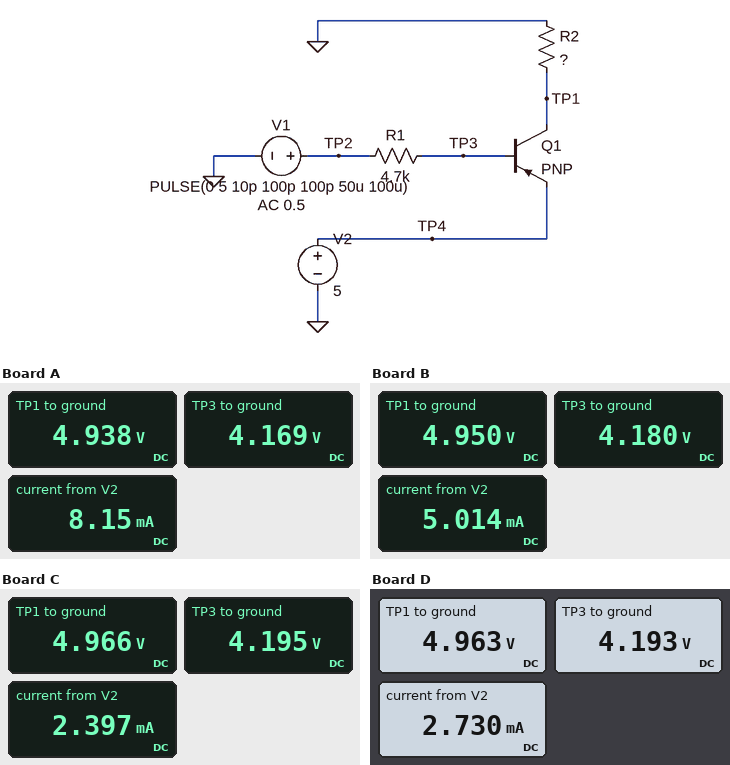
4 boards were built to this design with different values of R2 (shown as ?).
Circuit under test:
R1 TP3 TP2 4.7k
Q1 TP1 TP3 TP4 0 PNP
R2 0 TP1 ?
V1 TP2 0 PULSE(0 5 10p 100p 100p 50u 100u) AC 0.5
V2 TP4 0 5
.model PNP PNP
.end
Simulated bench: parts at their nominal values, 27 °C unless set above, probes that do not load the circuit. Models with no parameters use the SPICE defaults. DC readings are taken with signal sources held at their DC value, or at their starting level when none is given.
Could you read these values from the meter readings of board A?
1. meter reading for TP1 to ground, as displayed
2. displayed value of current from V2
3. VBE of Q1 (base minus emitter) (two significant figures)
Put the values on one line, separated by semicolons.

4.938 V; 8.15 mA; -830 mV
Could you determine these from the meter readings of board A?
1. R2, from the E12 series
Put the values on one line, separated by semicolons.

680 Ω
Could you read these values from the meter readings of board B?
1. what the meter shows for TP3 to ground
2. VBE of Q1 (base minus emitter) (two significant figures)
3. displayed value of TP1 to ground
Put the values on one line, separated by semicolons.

4.180 V; -820 mV; 4.950 V
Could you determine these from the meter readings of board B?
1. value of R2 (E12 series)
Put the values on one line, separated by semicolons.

1.2 kΩ
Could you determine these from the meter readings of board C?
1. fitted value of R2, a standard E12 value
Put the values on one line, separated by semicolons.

3.3 kΩ
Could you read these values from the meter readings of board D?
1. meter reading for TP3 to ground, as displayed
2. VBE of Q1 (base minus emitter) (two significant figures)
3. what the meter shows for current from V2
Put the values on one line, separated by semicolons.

4.193 V; -810 mV; 2.730 mA
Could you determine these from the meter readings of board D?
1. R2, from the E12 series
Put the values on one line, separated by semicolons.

2.7 kΩ
